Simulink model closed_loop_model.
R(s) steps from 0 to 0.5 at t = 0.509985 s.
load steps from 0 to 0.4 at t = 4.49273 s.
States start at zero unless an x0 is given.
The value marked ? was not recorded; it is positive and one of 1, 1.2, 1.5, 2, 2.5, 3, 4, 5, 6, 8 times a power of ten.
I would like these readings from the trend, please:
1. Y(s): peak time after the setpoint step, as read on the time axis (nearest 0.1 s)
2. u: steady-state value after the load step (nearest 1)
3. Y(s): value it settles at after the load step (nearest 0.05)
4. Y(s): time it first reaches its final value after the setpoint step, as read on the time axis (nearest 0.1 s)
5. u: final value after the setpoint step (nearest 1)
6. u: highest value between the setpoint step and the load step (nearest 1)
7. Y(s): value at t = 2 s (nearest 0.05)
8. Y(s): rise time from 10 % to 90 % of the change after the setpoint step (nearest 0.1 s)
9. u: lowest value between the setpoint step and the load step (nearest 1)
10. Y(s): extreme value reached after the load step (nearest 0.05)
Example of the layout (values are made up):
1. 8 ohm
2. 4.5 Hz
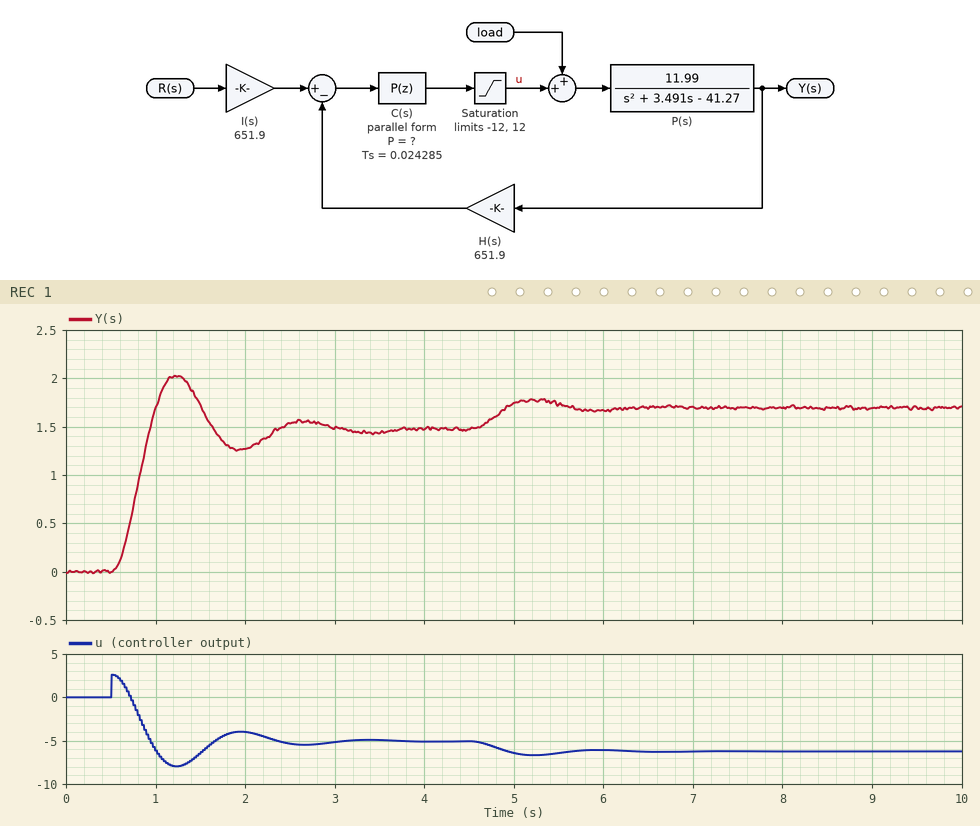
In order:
1. 1.2 s
2. -6
3. 1.70
4. 0.9 s
5. -5
6. 3
7. 1.25
8. 0.3 s
9. -8
10. 1.80
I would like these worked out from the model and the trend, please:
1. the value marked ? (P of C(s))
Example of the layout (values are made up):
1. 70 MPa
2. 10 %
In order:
1. 0.008
